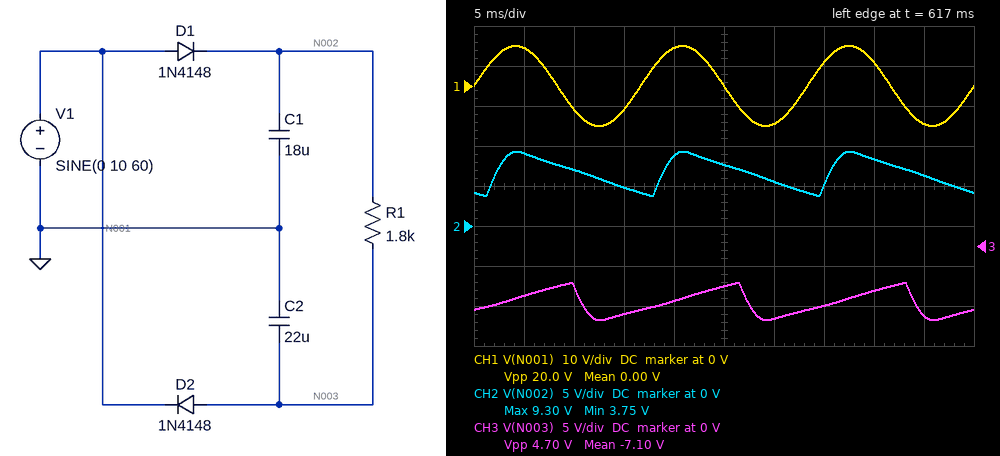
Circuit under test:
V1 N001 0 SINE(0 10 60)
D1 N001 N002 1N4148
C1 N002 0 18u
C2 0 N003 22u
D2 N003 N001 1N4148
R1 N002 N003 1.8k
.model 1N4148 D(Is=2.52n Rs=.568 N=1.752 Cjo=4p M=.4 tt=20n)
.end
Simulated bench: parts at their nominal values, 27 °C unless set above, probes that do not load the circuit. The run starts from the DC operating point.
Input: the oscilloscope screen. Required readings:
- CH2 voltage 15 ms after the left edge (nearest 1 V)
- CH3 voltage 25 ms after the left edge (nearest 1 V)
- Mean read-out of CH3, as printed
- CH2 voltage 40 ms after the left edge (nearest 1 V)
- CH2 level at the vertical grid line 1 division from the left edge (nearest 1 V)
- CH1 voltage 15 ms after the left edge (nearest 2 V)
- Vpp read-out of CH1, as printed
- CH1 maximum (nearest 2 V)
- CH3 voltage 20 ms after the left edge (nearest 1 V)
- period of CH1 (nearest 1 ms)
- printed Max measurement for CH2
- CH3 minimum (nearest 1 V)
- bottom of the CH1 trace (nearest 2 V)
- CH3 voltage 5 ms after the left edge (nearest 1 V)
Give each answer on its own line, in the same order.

5 V
-5 V
-7.10 V
8 V
9 V
-6 V
20.0 V
10 V
-7 V
17 ms
9.30 V
-9 V
-10 V
-6 V
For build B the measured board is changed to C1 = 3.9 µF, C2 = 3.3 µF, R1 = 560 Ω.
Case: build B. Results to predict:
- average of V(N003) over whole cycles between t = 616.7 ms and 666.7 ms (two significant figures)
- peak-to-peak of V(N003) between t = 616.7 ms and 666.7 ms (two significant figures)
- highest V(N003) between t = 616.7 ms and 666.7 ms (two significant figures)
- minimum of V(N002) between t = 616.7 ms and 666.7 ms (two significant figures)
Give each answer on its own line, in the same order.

-1.7 V
17 V
7.9 V
-7.3 V
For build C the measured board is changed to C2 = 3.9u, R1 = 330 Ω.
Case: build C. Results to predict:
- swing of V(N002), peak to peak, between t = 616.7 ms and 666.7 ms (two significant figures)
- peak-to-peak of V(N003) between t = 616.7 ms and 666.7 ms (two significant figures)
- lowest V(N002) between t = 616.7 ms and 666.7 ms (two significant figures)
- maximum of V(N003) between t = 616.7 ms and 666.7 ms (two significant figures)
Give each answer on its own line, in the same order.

12 V
18 V
-2.6 V
8.7 V
